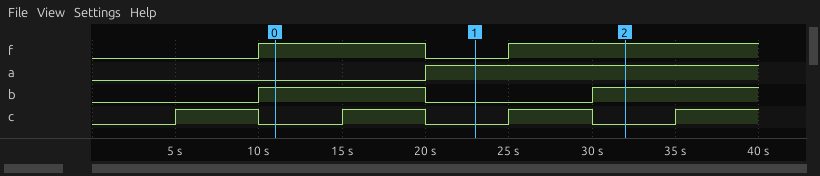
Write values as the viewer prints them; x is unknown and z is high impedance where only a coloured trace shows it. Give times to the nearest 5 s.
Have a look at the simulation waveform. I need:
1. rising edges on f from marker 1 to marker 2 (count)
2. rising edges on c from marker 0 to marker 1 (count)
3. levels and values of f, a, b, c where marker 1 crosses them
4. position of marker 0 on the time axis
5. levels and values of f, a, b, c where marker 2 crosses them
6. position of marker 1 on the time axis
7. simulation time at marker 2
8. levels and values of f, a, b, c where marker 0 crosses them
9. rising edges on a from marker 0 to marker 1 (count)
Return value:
1
1
f=0, a=1, b=0, c=0
10 s
f=1, a=1, b=1, c=0
25 s
30 s
f=1, a=0, b=1, c=0
1
